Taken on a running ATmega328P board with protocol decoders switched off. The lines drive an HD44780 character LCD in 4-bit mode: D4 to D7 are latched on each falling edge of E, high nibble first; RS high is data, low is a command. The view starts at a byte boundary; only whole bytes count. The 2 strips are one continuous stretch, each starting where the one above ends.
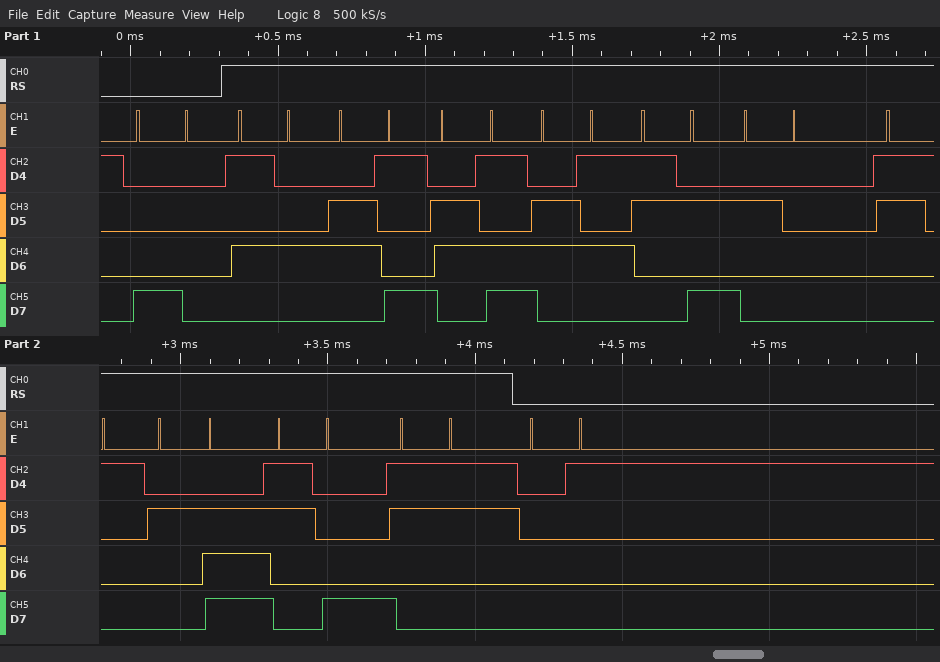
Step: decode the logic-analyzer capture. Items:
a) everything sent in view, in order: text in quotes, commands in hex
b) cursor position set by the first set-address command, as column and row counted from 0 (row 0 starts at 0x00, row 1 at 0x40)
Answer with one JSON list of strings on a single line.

["0x80 \"Time: 1.83\" 0x01", "column 0, row 0"]
